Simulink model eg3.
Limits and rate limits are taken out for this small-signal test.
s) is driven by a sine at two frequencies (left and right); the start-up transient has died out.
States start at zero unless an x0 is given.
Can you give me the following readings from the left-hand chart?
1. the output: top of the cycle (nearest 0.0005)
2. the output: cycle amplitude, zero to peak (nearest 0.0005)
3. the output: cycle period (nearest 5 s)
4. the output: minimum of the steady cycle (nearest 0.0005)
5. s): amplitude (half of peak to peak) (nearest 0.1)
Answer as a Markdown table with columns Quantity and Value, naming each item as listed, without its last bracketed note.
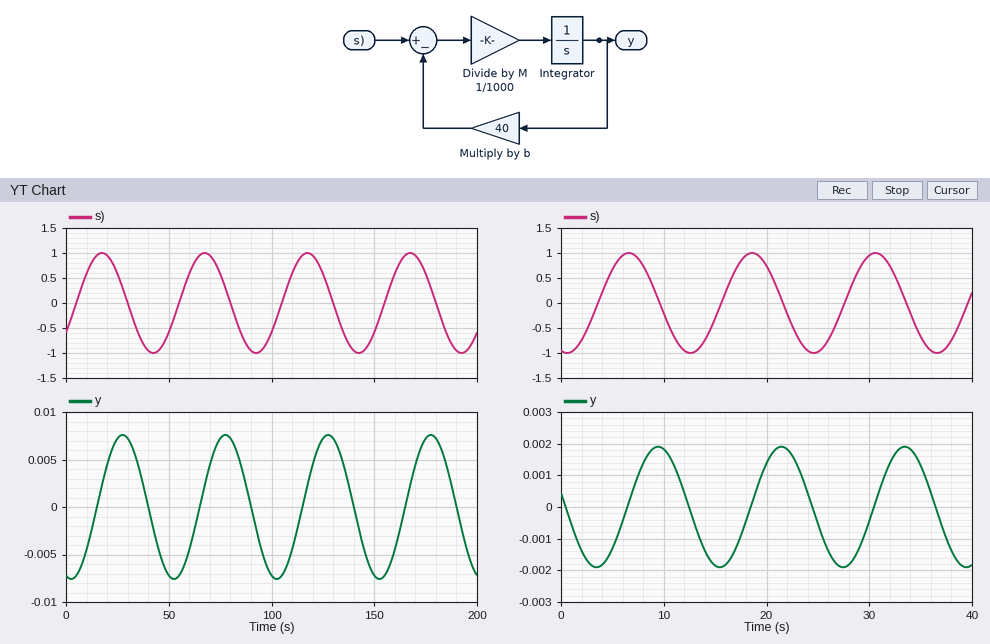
| Quantity | Value |
|---|---|
| the output: top of the cycle | 0.0075 |
| the output: cycle amplitude, zero to peak | 0.0075 |
| the output: cycle period | 50 s |
| the output: minimum of the steady cycle | -0.0075 |
| s): amplitude (half of peak to peak) | 1.0 |
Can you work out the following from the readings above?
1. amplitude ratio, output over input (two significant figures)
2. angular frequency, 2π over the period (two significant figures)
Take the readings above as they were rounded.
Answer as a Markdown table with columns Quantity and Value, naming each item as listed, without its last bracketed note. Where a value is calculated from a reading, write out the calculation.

| Quantity | Value |
|---|---|
| amplitude ratio, output over input | 0.0075 / 1 = 0.0075 |
| angular frequency, 2π over the period | 2π / 50 = 0.13 rad/s |
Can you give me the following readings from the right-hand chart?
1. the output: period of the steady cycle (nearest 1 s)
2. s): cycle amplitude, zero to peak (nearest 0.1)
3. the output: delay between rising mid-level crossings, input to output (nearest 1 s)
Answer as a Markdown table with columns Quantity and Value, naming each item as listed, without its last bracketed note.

| Quantity | Value |
|---|---|
| the output: period of the steady cycle | 12 s |
| s): cycle amplitude, zero to peak | 1.0 |
| the output: delay between rising mid-level crossings, input to output | 3 s |
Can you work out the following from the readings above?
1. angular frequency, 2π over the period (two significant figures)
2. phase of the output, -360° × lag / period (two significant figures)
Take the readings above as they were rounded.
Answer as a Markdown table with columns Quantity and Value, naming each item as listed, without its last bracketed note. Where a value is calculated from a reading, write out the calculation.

| Quantity | Value |
|---|---|
| angular frequency, 2π over the period | 2π / 12 = 0.52 rad/s |
| phase of the output, -360° × lag / period | -360 × 3 / 12 = -90° |
